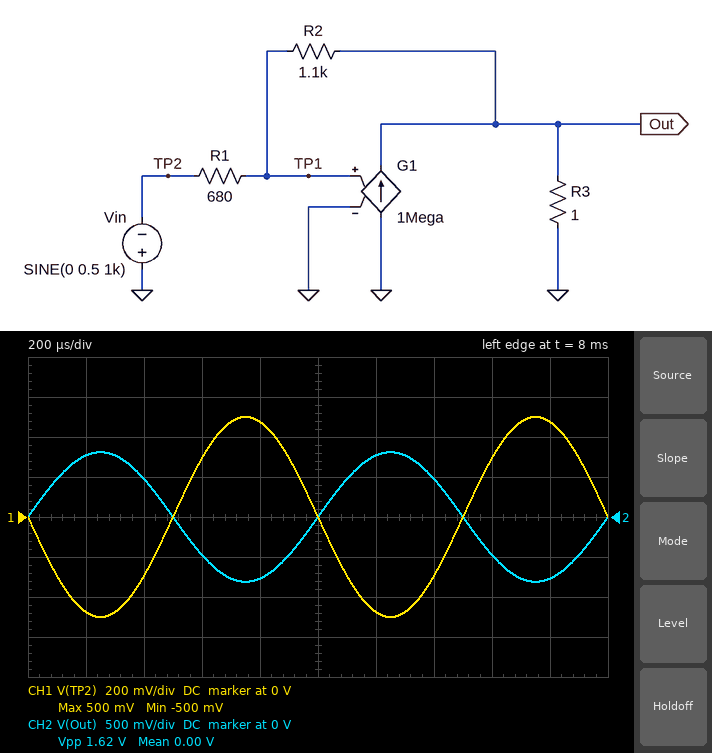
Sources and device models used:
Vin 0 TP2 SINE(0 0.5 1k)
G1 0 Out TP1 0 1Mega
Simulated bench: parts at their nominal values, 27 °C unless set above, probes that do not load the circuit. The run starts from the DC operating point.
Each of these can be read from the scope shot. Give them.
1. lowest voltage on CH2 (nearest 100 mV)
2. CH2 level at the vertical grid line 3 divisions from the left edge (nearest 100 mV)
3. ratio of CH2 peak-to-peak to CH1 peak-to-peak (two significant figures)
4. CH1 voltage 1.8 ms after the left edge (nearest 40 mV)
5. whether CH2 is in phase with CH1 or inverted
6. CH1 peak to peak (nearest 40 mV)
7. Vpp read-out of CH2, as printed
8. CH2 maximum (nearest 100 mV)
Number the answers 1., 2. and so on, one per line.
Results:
1. -800 mV
2. -500 mV
3. 1.6
4. 480 mV
5. inverted
6. 1.00 V
7. 1.62 V
8. 800 mV
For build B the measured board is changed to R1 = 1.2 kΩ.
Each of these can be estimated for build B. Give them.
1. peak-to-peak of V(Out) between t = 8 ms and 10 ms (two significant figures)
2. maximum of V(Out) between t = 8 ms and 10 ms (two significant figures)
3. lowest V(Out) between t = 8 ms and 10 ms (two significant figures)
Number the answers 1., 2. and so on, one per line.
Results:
1. 920 mV
2. 460 mV
3. -460 mV
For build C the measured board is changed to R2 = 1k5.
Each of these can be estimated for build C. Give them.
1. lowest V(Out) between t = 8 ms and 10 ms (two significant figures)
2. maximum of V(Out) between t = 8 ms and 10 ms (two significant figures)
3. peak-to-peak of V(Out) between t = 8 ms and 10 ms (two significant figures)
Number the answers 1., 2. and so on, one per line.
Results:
1. -1.1 V
2. 1.1 V
3. 2.2 V
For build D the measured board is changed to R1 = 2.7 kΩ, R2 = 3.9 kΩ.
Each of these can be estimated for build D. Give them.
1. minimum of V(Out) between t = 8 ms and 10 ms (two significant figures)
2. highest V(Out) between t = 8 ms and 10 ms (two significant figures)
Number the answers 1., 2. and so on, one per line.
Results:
1. -720 mV
2. 720 mV
